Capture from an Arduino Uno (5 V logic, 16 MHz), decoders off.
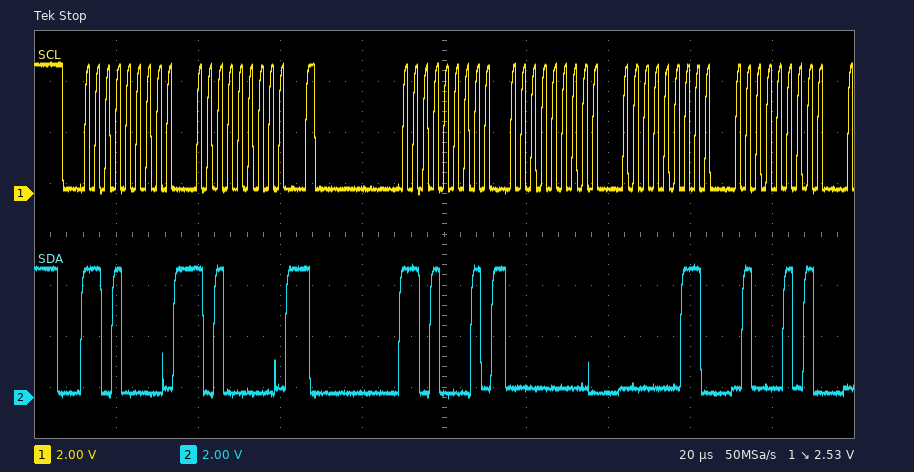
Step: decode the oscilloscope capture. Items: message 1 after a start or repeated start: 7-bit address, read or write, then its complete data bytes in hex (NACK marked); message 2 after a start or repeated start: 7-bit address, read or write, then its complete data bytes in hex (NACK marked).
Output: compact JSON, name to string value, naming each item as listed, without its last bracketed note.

{"message 1 after a start or repeated start: 7-bit address, read or write, then its complete data bytes in hex": "0x68 write: A0", "message 2 after a start or repeated start: 7-bit address, read or write, then its complete data bytes in hex": "0x68 read: 00 03 45"}
